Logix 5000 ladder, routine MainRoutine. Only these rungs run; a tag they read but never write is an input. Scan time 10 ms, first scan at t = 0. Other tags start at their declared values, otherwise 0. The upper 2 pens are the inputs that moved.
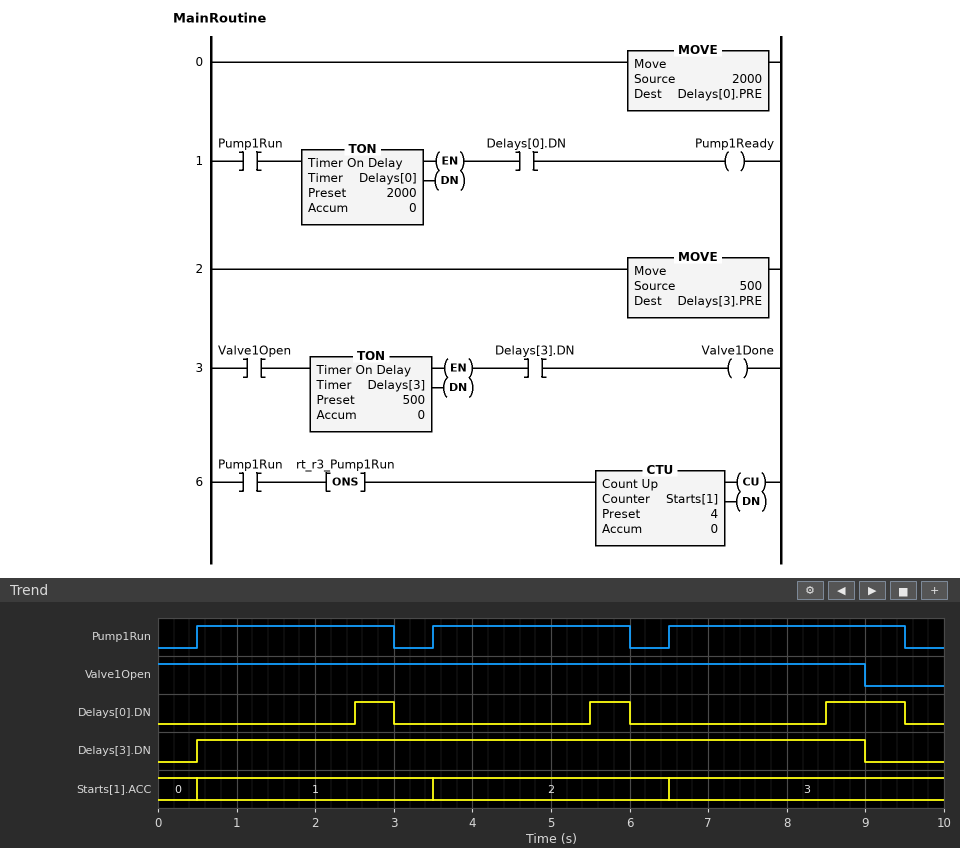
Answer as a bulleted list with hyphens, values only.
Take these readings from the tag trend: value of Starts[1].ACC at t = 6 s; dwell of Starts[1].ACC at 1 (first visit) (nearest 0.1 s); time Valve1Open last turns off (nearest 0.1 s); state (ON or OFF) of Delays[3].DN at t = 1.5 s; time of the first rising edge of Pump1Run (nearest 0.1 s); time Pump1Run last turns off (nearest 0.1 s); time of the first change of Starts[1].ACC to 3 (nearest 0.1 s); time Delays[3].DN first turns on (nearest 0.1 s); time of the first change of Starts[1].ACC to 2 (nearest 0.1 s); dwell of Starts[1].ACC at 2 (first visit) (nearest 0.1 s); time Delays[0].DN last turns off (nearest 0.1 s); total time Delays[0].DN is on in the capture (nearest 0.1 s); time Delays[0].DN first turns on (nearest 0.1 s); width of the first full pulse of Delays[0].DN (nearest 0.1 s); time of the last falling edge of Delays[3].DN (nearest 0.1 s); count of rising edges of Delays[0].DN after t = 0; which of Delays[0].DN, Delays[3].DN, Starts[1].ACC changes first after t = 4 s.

- 2
- 3.0 s
- 9.0 s
- ON
- 0.5 s
- 9.5 s
- 6.5 s
- 0.5 s
- 3.5 s
- 3.0 s
- 9.5 s
- 2.0 s
- 2.5 s
- 0.5 s
- 9.0 s
- 3
- Delays[0].DN
